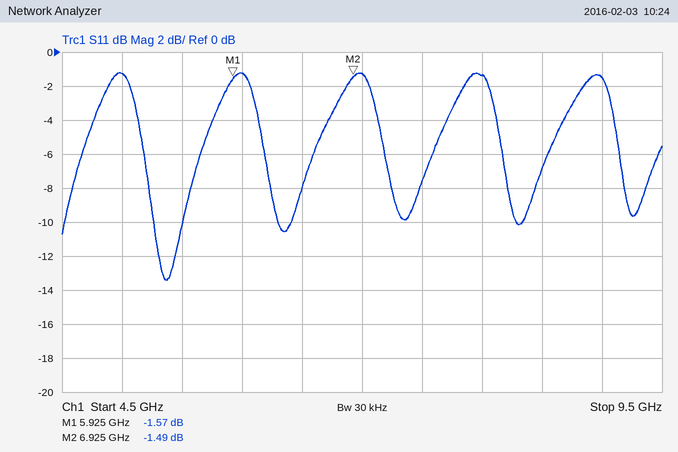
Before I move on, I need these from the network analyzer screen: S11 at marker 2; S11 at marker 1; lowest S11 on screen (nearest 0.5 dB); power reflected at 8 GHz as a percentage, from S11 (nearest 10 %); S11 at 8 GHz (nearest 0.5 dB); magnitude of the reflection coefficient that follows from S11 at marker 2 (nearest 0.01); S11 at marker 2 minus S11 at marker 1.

-1.49 dB
-1.57 dB
-13.5 dB
70 %
-1.5 dB
0.84
0.08 dB
